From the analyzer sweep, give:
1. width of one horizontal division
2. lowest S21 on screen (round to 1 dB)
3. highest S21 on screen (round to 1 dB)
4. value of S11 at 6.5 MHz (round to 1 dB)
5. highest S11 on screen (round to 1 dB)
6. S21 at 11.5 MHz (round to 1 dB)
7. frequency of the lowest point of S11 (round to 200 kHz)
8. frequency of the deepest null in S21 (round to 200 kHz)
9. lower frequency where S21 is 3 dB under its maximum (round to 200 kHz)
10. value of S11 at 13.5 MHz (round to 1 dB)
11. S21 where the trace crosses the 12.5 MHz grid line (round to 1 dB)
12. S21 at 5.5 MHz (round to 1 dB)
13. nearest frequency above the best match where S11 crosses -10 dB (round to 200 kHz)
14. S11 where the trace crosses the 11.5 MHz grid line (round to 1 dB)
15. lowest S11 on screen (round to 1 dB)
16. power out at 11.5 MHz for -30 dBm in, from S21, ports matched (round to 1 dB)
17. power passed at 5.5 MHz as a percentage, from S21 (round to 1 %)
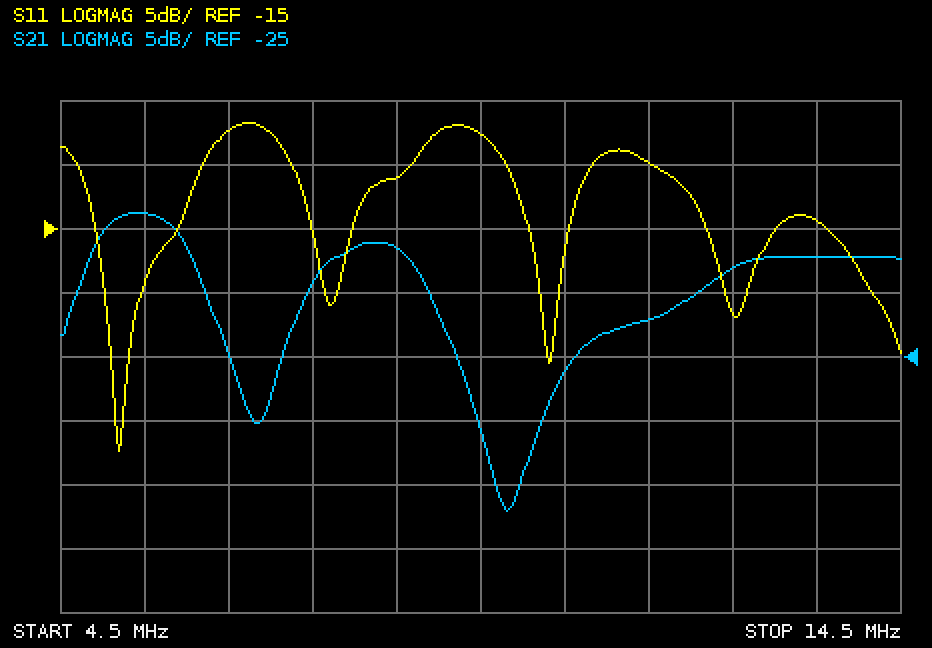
1 MHz
-37 dB
-14 dB
-7 dB
-7 dB
-22 dB
5.2 MHz
9.8 MHz
4.8 MHz
-14 dB
-18 dB
-14 dB
6.2 MHz
-10 dB
-32 dB
-52 dBm
4 %
